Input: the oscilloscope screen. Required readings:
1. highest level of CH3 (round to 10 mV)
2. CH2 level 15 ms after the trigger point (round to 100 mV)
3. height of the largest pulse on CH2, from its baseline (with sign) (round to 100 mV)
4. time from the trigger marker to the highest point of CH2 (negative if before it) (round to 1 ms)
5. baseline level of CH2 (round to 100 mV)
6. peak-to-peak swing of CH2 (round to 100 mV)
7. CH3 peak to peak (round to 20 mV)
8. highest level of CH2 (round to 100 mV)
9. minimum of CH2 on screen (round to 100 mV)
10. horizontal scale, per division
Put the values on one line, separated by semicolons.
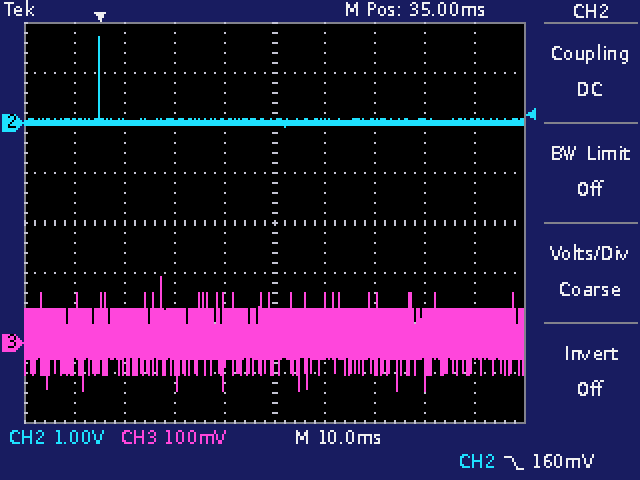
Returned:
130 mV; 0.0 V; +1.7 V; 0 ms; 0.0 V; 1.8 V; 220 mV; 1.7 V; -100 mV; 10 ms
